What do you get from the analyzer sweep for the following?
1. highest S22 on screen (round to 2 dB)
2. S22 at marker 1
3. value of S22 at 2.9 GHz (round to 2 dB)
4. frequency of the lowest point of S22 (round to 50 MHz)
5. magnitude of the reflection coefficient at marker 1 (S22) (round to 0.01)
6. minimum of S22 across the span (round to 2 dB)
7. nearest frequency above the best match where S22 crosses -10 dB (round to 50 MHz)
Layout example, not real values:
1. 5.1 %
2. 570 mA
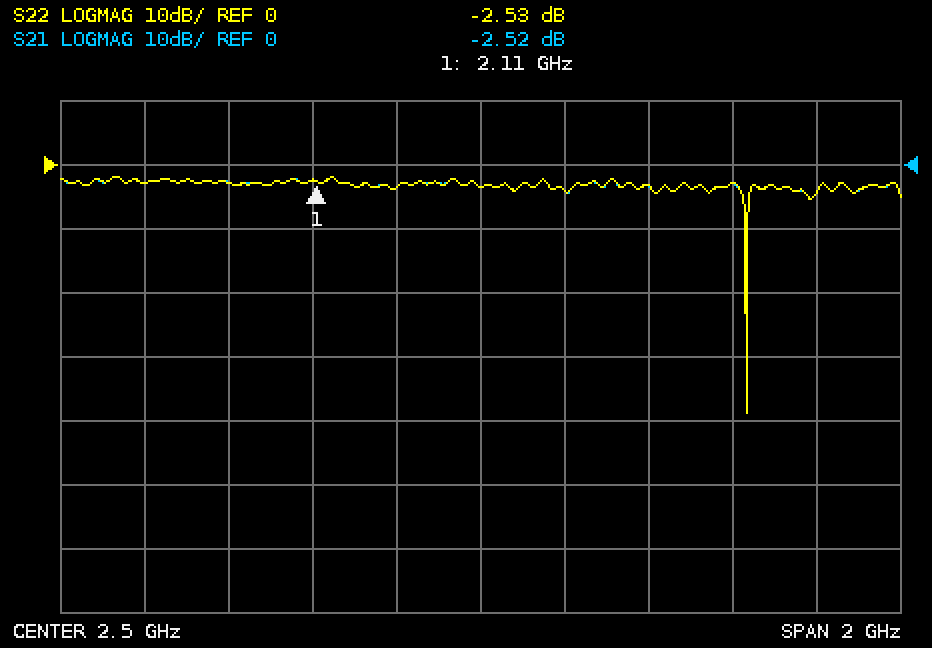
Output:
1. -2 dB
2. -2.53 dB
3. -4 dB
4. 3.15 GHz
5. 0.75
6. -38 dB
7. 3.15 GHz
